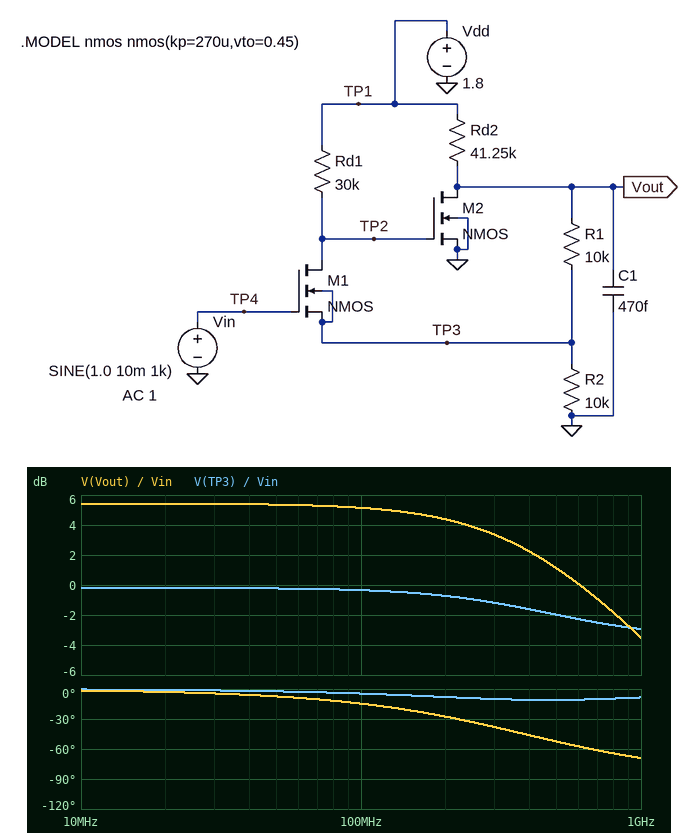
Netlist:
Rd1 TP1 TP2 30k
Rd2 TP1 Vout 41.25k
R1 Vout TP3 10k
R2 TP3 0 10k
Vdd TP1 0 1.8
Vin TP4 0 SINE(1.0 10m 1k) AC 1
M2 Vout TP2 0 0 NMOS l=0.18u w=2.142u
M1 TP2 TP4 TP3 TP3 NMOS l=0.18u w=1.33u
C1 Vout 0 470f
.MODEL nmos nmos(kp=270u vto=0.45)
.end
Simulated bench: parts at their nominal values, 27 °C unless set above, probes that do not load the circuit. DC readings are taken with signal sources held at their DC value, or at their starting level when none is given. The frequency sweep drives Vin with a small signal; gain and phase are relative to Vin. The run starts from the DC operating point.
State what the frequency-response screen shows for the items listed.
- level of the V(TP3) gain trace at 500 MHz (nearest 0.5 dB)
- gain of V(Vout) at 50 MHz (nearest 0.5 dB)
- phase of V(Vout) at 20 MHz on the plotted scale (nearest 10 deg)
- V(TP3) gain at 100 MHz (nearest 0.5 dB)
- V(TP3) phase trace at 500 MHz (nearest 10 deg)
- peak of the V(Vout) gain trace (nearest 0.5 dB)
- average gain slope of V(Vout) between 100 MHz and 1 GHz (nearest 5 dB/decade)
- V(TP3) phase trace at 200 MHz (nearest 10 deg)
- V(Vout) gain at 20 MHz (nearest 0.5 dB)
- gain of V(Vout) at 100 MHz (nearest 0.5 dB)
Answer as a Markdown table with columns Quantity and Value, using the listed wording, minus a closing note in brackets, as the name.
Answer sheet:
| Quantity | Value |
|---|---|
| level of the V(TP3) gain trace at 500 MHz | -2.0 dB |
| gain of V(Vout) at 50 MHz | 5.5 dB |
| phase of V(Vout) at 20 MHz on the plotted scale | 0 deg |
| V(TP3) gain at 100 MHz | -0.5 dB |
| V(TP3) phase trace at 500 MHz | -10 deg |
| peak of the V(Vout) gain trace | 5.5 dB |
| average gain slope of V(Vout) between 100 MHz and 1 GHz | -10 dB/decade |
| V(TP3) phase trace at 200 MHz | -10 deg |
| V(Vout) gain at 20 MHz | 5.5 dB |
| gain of V(Vout) at 100 MHz | 5.0 dB |
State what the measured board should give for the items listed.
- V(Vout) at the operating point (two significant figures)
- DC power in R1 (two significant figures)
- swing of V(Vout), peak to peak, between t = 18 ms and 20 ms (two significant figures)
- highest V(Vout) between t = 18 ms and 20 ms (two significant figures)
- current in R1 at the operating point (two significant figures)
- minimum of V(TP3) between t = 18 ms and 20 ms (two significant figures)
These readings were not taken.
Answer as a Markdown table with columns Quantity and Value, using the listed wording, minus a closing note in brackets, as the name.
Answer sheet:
| Quantity | Value |
|---|---|
| V(Vout) at the operating point | 300 mV |
| DC power in R1 | 210 nW |
| swing of V(Vout), peak to peak, between t = 18 ms and 20 ms | 37 mV |
| highest V(Vout) between t = 18 ms and 20 ms | 320 mV |
| current in R1 at the operating point | 4.6 µA |
| minimum of V(TP3) between t = 18 ms and 20 ms | 340 mV |
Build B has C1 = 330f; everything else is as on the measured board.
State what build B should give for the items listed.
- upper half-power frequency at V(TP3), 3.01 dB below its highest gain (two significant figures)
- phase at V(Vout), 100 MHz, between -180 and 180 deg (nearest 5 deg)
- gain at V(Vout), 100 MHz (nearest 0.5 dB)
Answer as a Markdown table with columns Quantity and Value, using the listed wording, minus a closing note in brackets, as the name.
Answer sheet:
| Quantity | Value |
|---|---|
| upper half-power frequency at V(TP3), 3.01 dB below its highest gain | 2.0 GHz |
| phase at V(Vout), 100 MHz, between -180 and 180 deg | -10 deg |
| gain at V(Vout), 100 MHz | 5.5 dB |
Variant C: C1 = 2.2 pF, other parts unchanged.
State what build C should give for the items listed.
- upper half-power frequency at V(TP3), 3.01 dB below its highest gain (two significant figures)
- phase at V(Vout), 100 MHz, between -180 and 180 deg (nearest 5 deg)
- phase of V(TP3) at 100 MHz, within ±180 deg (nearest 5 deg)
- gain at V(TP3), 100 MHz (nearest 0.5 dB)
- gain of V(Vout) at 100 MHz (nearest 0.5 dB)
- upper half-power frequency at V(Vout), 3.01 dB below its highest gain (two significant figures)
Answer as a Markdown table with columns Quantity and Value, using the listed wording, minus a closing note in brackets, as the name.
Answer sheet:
| Quantity | Value |
|---|---|
| upper half-power frequency at V(TP3), 3.01 dB below its highest gain | 300 MHz |
| phase at V(Vout), 100 MHz, between -180 and 180 deg | -50 deg |
| phase of V(TP3) at 100 MHz, within ±180 deg | -10 deg |
| gain at V(TP3), 100 MHz | -2.0 dB |
| gain of V(Vout) at 100 MHz | 1.5 dB |
| upper half-power frequency at V(Vout), 3.01 dB below its highest gain | 82 MHz |
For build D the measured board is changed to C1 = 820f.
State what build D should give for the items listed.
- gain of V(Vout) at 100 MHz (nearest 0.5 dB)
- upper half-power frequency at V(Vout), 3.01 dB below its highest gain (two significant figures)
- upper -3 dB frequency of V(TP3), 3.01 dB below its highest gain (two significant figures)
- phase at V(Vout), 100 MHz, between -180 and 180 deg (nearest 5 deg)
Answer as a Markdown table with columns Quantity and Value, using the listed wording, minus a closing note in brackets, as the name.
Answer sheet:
| Quantity | Value |
|---|---|
| gain of V(Vout) at 100 MHz | 4.5 dB |
| upper half-power frequency at V(Vout), 3.01 dB below its highest gain | 220 MHz |
| upper -3 dB frequency of V(TP3), 3.01 dB below its highest gain | 810 MHz |
| phase at V(Vout), 100 MHz, between -180 and 180 deg | -25 deg |
